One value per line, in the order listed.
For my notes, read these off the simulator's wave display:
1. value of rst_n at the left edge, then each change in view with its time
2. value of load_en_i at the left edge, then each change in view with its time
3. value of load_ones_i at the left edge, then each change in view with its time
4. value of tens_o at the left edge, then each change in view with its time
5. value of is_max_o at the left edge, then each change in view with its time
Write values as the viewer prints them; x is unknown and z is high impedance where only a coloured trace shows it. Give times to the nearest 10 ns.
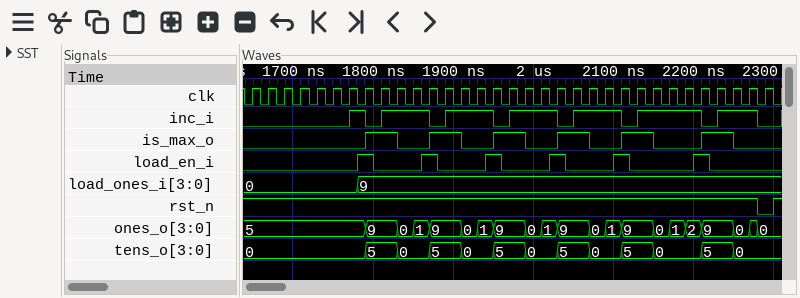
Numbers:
1, 0 at 2280 ns, 1 at 2300 ns
0, 1 at 1780 ns, 0 at 1800 ns, 1 at 1860 ns, 0 at 1880 ns, 1 at 1940 ns, 0 at 1960 ns, 1 at 2020 ns, 0 at 2040 ns, 1 at 2100 ns, 0 at 2120 ns, 1 at 2200 ns, 0 at 2220 ns
0, 9 at 1780 ns
0, 5 at 1790 ns, 0 at 1830 ns, 5 at 1870 ns, 0 at 1910 ns, 5 at 1950 ns, 0 at 1990 ns, 5 at 2030 ns, 0 at 2070 ns, 5 at 2110 ns, 0 at 2150 ns, 5 at 2210 ns, 0 at 2250 ns
0, 1 at 1790 ns, 0 at 1830 ns, 1 at 1870 ns, 0 at 1910 ns, 1 at 1950 ns, 0 at 1990 ns, 1 at 2030 ns, 0 at 2070 ns, 1 at 2110 ns, 0 at 2150 ns, 1 at 2210 ns, 0 at 2250 ns
